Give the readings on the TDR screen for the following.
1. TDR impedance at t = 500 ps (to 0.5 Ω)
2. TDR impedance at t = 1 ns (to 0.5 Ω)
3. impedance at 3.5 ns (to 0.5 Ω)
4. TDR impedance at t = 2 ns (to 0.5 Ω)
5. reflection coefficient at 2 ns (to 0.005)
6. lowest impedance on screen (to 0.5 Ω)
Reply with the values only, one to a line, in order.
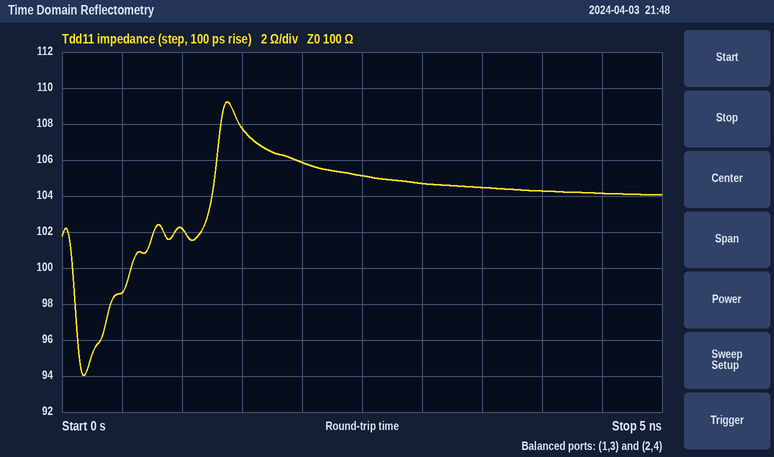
98.5 Ω
102.0 Ω
104.5 Ω
106.0 Ω
+0.030
94.0 Ω
